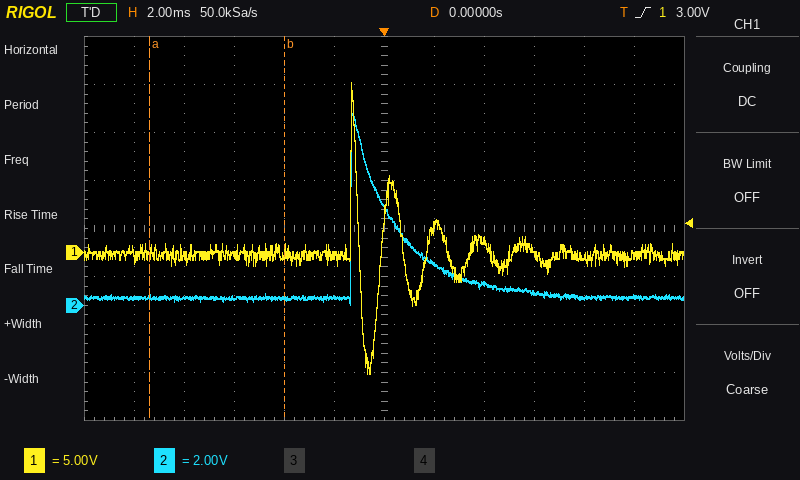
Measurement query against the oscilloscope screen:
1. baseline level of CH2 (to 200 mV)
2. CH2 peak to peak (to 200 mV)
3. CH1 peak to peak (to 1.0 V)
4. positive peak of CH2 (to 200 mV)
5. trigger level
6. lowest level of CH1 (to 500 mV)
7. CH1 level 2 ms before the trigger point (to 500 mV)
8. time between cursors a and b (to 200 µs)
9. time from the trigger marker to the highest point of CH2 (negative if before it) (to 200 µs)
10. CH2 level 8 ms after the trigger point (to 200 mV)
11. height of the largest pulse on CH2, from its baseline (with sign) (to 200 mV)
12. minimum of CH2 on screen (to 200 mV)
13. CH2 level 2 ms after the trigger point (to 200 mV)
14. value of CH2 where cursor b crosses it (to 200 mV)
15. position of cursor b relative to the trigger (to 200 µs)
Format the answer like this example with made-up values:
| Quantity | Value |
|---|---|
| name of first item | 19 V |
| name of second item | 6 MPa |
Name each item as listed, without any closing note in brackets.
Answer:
| Quantity | Value |
|---|---|
| baseline level of CH2 | 400 mV |
| CH2 peak to peak | 8.0 V |
| CH1 peak to peak | 30.0 V |
| positive peak of CH2 | 8.0 V |
| trigger level | 3.00 V |
| lowest level of CH1 | -12.5 V |
| CH1 level 2 ms before the trigger point | -500 mV |
| time between cursors a and b | 5.4 ms |
| time from the trigger marker to the highest point of CH2 (negative if before it) | -1.2 ms |
| CH2 level 8 ms after the trigger point | 400 mV |
| height of the largest pulse on CH2, from its baseline (with sign) | +7.6 V |
| minimum of CH2 on screen | 0.0 V |
| CH2 level 2 ms after the trigger point | 1.8 V |
| value of CH2 where cursor b crosses it | 200 mV |
| position of cursor b relative to the trigger | -4.0 ms |
